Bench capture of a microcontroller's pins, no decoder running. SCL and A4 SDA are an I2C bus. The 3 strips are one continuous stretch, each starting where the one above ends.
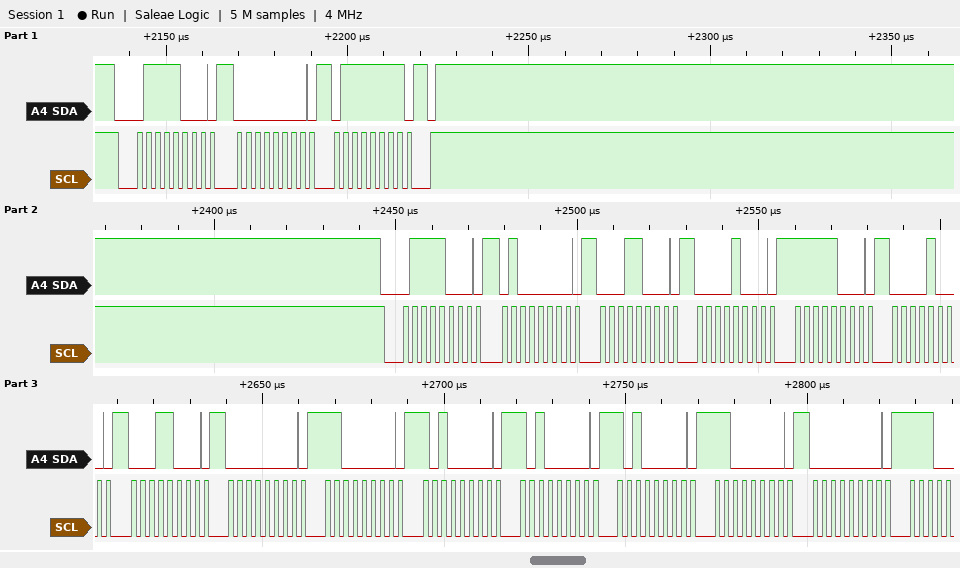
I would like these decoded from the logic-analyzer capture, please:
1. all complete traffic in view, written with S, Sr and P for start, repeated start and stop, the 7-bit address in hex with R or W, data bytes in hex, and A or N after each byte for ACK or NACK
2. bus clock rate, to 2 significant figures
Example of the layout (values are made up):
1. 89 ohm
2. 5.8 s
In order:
1. S 3CW A 00 A 7F A P S 3CW A 40 A 18 A 08 A F8 A 08 A 18 A 00 A C0 A A0 A A0 A A0 A C0 A 00 A
2. 400 kHz
